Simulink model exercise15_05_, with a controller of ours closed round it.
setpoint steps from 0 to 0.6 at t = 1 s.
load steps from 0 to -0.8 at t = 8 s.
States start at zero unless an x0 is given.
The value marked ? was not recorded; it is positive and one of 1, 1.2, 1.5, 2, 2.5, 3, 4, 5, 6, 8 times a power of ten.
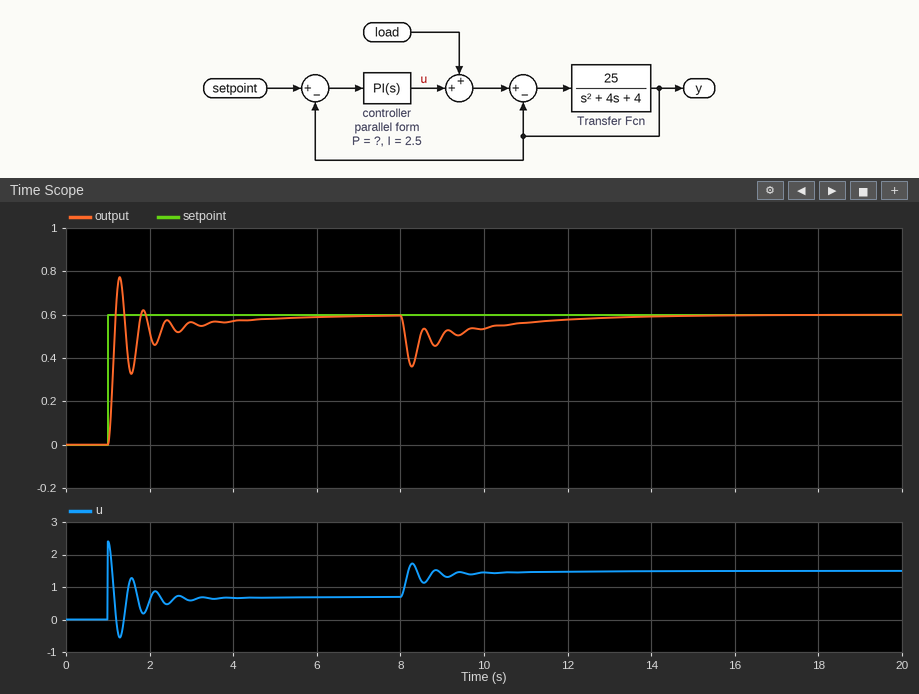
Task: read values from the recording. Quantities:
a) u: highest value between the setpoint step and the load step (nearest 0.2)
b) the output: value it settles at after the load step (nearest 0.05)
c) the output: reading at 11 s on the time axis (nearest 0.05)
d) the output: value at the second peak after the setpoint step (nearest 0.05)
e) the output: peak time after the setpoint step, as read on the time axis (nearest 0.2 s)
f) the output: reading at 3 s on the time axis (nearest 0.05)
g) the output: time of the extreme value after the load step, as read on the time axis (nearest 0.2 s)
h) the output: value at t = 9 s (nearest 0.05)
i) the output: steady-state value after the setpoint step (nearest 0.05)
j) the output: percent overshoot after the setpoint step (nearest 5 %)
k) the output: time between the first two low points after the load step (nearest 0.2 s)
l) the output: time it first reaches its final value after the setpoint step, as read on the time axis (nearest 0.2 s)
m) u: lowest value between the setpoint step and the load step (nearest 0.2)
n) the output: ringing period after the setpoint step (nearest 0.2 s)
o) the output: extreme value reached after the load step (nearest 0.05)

2.4
0.60
0.55
0.60
1.2 s
0.55
8.2 s
0.50
0.60
30 %
0.6 s
1.2 s
-0.6
0.6 s
0.35
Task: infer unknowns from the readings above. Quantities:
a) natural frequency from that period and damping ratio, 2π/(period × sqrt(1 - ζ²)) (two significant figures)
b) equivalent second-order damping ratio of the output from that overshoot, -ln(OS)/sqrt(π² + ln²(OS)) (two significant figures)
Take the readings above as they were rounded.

11 rad/s
0.36
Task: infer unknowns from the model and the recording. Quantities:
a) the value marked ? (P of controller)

4
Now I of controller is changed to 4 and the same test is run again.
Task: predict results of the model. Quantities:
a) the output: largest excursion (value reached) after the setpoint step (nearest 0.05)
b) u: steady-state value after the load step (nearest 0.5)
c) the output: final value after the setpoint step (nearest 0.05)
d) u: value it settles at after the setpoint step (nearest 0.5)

0.80
1.5
0.60
0.5
